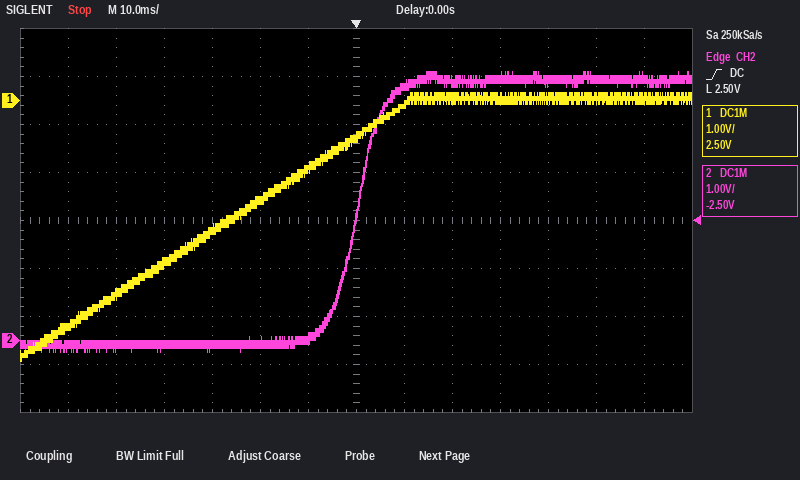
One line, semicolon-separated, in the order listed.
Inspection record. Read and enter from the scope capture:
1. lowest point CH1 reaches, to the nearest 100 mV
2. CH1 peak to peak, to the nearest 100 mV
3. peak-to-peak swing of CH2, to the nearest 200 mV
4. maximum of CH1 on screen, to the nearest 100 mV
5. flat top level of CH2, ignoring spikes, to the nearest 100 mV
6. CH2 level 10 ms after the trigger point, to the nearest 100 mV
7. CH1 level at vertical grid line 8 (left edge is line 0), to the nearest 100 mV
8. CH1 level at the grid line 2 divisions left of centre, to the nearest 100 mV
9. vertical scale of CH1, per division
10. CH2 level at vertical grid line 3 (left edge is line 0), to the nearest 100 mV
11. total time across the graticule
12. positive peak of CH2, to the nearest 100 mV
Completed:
-5.4 V; 5.6 V; 5.8 V; 200 mV; 5.4 V; 5.3 V; -100 mV; -2.1 V; 1 V; -100 mV; 140 ms; 5.6 V
